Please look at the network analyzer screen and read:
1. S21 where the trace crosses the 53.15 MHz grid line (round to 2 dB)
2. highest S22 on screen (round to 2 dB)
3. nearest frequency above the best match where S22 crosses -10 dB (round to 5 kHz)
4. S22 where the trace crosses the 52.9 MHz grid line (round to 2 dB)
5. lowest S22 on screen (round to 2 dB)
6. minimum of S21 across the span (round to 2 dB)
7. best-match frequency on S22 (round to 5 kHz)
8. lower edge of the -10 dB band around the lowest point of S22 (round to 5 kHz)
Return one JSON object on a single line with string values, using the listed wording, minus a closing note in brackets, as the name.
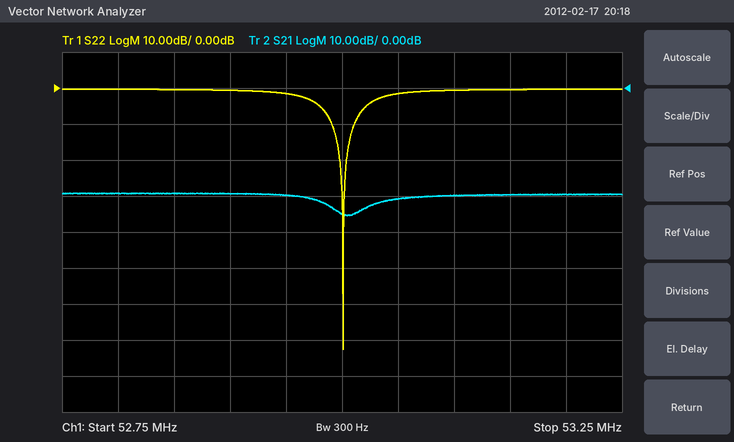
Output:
{"S21 where the trace crosses the 53.15 MHz grid line": "-30 dB", "highest S22 on screen": "0 dB", "nearest frequency above the best match where S22 crosses -10 dB": "53.010 MHz", "S22 where the trace crosses the 52.9 MHz grid line": "0 dB", "lowest S22 on screen": "-72 dB", "minimum of S21 across the span": "-36 dB", "best-match frequency on S22": "53.000 MHz", "lower edge of the -10 dB band around the lowest point of S22": "52.990 MHz"}
